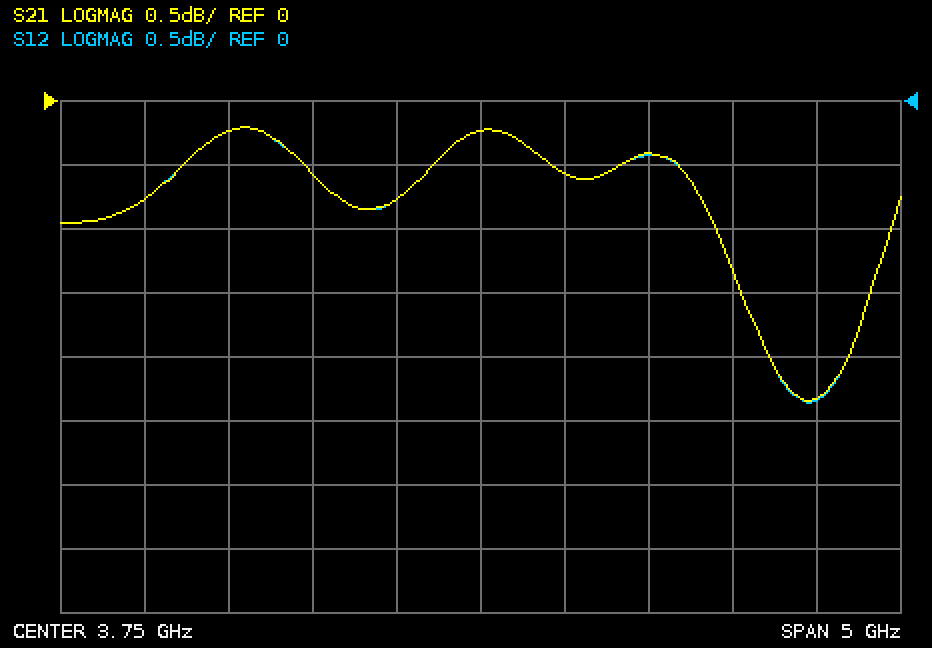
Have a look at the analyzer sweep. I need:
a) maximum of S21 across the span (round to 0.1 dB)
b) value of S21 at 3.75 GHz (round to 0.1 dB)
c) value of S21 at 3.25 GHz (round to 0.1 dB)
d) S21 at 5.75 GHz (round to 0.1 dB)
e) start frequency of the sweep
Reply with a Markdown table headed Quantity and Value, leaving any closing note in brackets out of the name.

| Quantity | Value |
|---|---|
| maximum of S21 across the span | -0.2 dB |
| value of S21 at 3.75 GHz | -0.2 dB |
| value of S21 at 3.25 GHz | -0.8 dB |
| S21 at 5.75 GHz | -2.3 dB |
| start frequency of the sweep | 1.25 GHz |
